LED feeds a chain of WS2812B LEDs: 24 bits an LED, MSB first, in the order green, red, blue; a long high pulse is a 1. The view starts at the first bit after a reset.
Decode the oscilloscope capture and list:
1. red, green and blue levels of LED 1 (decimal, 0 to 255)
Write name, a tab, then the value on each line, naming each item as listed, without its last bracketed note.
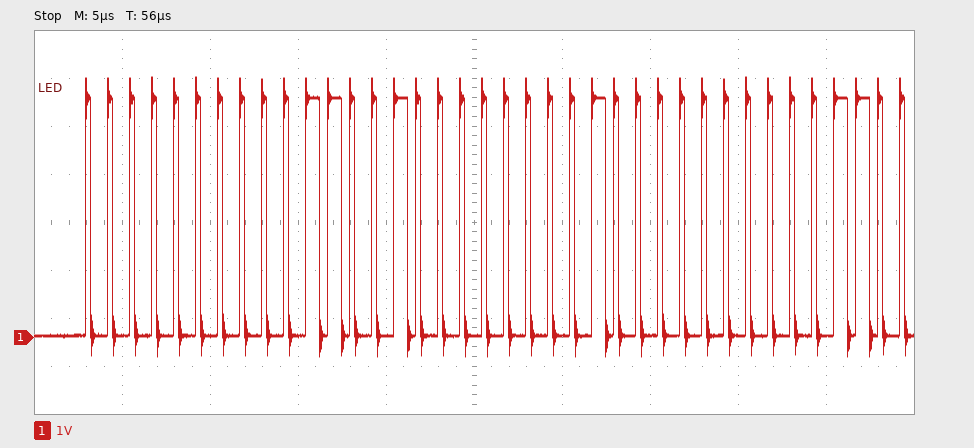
red, green and blue levels of LED 1	50, 0, 1
